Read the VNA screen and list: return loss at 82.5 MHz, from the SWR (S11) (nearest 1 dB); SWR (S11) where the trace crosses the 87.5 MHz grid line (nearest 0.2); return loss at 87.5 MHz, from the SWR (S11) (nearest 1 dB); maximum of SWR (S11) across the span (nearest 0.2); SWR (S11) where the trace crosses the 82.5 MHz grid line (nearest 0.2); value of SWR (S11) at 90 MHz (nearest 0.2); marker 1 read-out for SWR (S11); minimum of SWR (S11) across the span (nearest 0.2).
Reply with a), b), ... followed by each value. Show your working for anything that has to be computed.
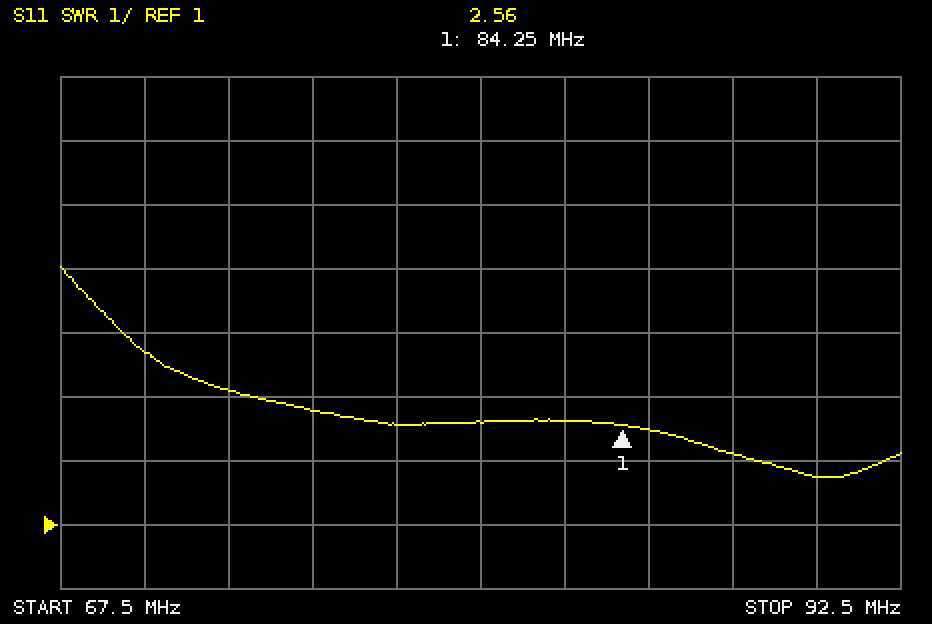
a) −20 log10((2.6 − 1)/(2.6 + 1)) ≈ 7 dB
b) 2.2
c) −20 log10((2.2 − 1)/(2.2 + 1)) ≈ 9 dB
d) 5.0
e) 2.6
f) 1.8
g) 2.56
h) 1.8
